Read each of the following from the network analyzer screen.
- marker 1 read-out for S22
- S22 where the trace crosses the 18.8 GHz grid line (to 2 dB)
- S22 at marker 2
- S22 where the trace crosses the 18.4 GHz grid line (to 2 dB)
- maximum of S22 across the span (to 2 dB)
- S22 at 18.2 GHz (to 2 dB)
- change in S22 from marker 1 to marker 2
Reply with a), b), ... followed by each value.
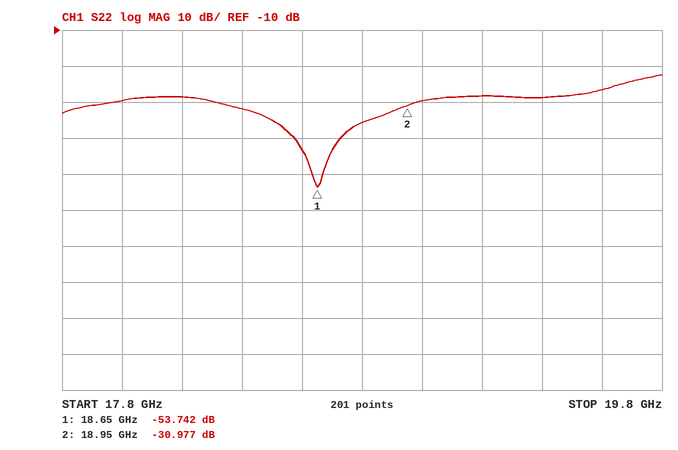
a) -53.742 dB
b) -36 dB
c) -30.977 dB
d) -32 dB
e) -22 dB
f) -28 dB
g) 22.765 dB
